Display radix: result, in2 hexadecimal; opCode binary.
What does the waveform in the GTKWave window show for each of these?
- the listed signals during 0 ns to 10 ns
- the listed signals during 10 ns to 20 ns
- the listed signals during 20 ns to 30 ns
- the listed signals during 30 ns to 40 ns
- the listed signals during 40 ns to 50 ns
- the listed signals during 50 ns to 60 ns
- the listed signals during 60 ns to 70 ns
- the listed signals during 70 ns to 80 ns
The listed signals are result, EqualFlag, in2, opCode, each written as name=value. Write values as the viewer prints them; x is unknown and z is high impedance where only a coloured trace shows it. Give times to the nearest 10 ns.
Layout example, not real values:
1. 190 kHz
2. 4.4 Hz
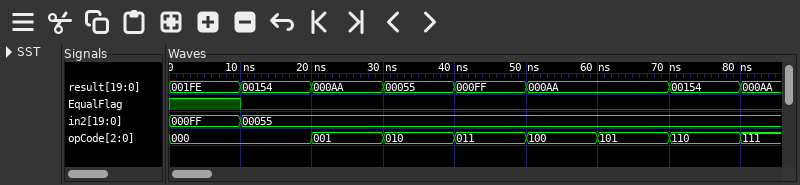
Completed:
1. result=001FE, EqualFlag=1, in2=000FF, opCode=000
2. result=00154, EqualFlag=0, in2=00055, opCode=000
3. result=000AA, EqualFlag=0, in2=00055, opCode=001
4. result=00055, EqualFlag=0, in2=00055, opCode=010
5. result=000FF, EqualFlag=0, in2=00055, opCode=011
6. result=000AA, EqualFlag=0, in2=00055, opCode=100
7. result=000AA, EqualFlag=0, in2=00055, opCode=101
8. result=00154, EqualFlag=0, in2=00055, opCode=110
